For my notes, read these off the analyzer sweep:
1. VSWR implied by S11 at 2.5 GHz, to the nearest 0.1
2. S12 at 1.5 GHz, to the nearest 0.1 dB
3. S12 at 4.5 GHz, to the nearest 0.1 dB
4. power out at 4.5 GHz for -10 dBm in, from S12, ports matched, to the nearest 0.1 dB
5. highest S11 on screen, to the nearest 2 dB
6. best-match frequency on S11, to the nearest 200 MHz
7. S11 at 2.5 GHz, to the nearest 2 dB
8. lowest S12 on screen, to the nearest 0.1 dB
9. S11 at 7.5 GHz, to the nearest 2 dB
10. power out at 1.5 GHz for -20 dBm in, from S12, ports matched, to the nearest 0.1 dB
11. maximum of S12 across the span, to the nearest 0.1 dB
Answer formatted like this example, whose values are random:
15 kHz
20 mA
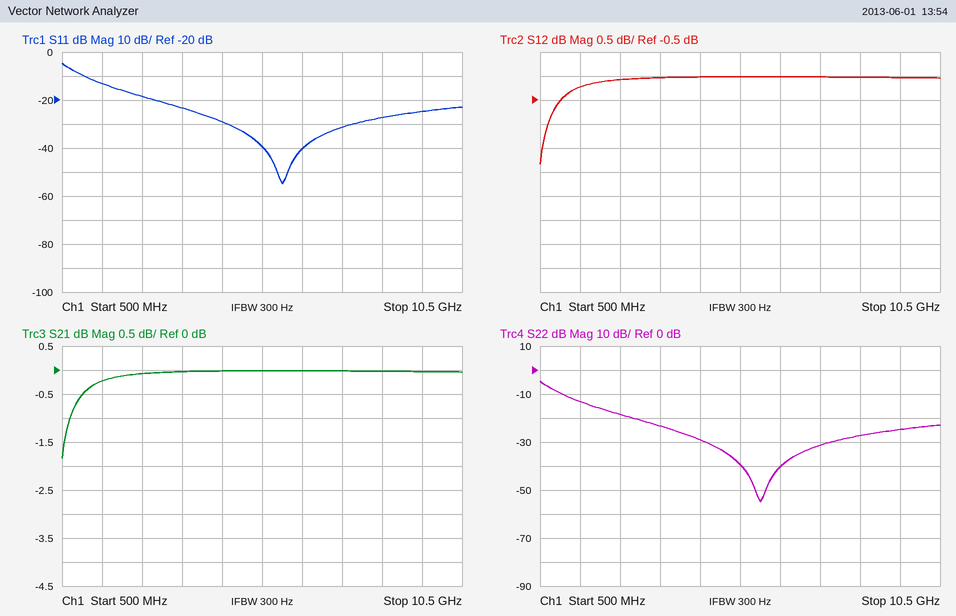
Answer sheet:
1.3
-0.2 dB
0.0 dB
-10.0 dBm
-4 dB
6.0 GHz
-18 dB
-1.8 dB
-32 dB
-20.2 dBm
0.0 dB
